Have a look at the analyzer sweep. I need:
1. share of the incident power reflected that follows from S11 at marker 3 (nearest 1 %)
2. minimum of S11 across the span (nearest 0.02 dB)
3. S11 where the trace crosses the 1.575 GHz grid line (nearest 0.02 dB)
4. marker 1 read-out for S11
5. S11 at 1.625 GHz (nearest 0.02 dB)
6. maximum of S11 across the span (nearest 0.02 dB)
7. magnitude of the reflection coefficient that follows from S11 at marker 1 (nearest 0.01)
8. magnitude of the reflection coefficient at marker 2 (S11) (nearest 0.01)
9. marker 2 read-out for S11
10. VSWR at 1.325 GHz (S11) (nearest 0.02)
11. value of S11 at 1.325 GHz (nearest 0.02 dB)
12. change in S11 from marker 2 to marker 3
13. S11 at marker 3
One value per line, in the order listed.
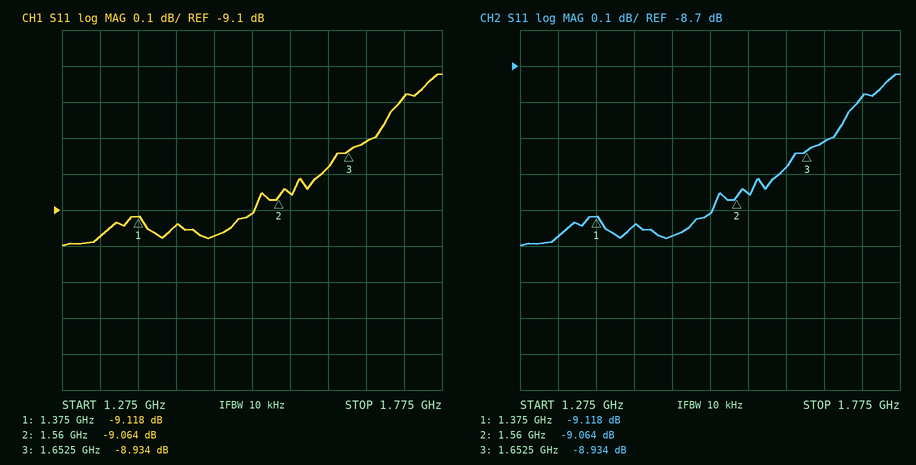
13 %
-9.20 dB
-9.06 dB
-9.118 dB
-8.98 dB
-8.72 dB
0.35
0.35
-9.064 dB
2.06
-9.18 dB
0.130 dB
-8.934 dB
